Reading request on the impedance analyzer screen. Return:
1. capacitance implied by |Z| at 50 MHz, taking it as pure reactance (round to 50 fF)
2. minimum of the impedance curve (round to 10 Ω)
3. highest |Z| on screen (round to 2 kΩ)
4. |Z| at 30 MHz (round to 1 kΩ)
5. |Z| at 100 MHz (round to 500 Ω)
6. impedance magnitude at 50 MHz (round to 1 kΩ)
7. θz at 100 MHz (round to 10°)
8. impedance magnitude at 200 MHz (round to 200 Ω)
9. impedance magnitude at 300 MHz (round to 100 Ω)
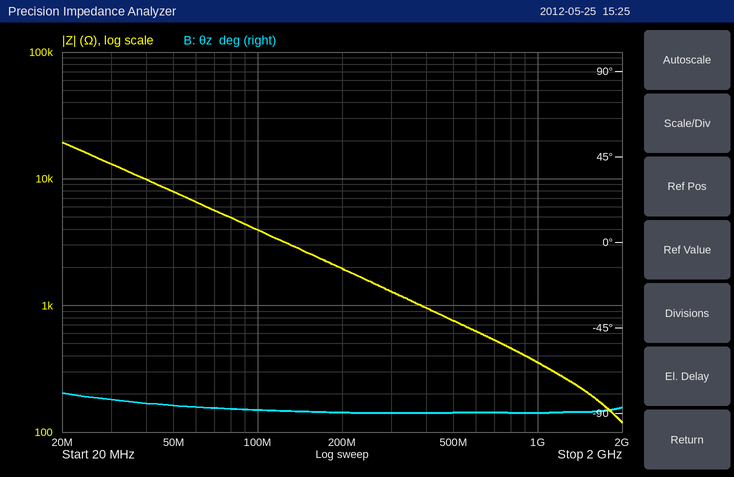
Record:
400 fF
120 Ω
20 kΩ
13 kΩ
4.0 kΩ
8 kΩ
-90°
2.0 kΩ
1.3 kΩ
